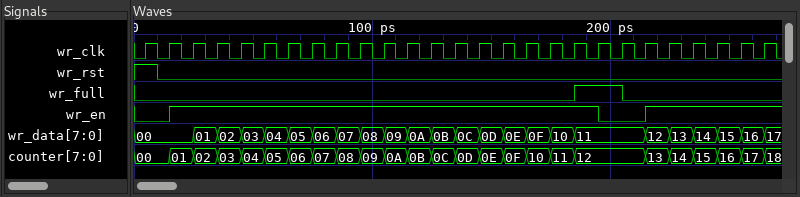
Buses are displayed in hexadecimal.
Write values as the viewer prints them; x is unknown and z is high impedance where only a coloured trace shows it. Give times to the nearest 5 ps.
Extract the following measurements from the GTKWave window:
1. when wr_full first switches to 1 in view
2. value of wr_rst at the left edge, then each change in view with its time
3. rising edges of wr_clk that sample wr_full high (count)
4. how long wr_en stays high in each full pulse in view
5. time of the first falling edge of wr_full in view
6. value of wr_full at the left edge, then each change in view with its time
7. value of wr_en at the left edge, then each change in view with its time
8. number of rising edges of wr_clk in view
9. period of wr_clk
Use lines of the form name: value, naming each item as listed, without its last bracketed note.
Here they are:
when wr_full first switches to 1 in view: 185 ps
value of wr_rst at the left edge, then each change in view with its time: 1, 0 at 10 ps
rising edges of wr_clk that sample wr_full high: 2
how long wr_en stays high in each full pulse in view: 180 ps
time of the first falling edge of wr_full in view: 205 ps
value of wr_full at the left edge, then each change in view with its time: 0, 1 at 185 ps, 0 at 205 ps
value of wr_en at the left edge, then each change in view with its time: 0, 1 at 15 ps, 0 at 195 ps, 1 at 215 ps
number of rising edges of wr_clk in view: 27
period of wr_clk: 10 ps
